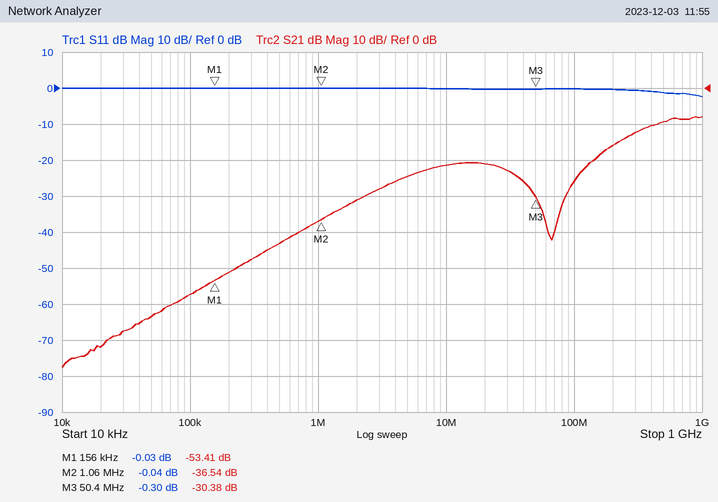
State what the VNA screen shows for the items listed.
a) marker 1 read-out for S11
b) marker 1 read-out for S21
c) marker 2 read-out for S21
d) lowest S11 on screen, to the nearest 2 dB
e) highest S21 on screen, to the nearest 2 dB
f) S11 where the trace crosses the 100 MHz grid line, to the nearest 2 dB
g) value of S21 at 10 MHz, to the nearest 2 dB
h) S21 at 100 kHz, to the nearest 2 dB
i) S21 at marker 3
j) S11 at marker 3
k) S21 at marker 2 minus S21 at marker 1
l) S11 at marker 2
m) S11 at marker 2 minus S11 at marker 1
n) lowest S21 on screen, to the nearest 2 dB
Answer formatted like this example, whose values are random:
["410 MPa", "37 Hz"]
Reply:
["-0.03 dB", "-53.41 dB", "-36.54 dB", "-2 dB", "-8 dB", "0 dB", "-22 dB", "-58 dB", "-30.38 dB", "-0.30 dB", "16.87 dB", "-0.04 dB", "-0.01 dB", "-78 dB"]
